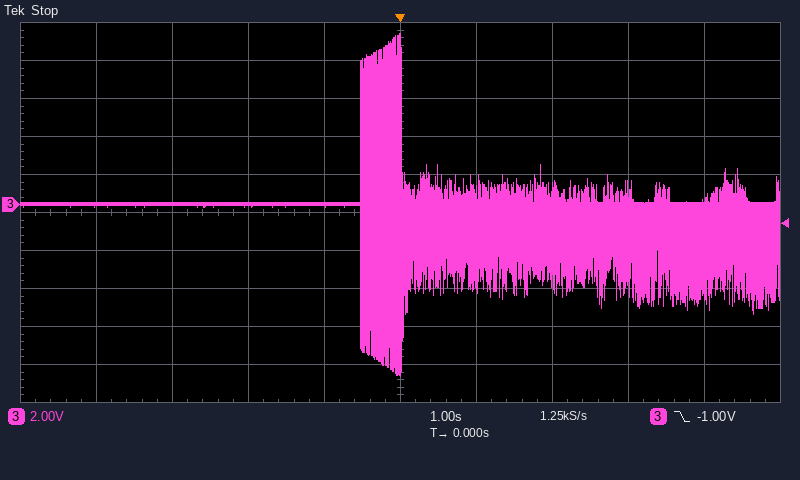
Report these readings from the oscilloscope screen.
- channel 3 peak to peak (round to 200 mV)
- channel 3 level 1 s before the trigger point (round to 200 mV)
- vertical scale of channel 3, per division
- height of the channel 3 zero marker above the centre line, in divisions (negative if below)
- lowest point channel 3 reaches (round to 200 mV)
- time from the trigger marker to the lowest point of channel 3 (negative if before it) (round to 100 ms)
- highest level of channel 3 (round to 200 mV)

18.0 V
0.0 V
2 V
+0.2 div
-9.0 V
0.0 s
9.0 V
